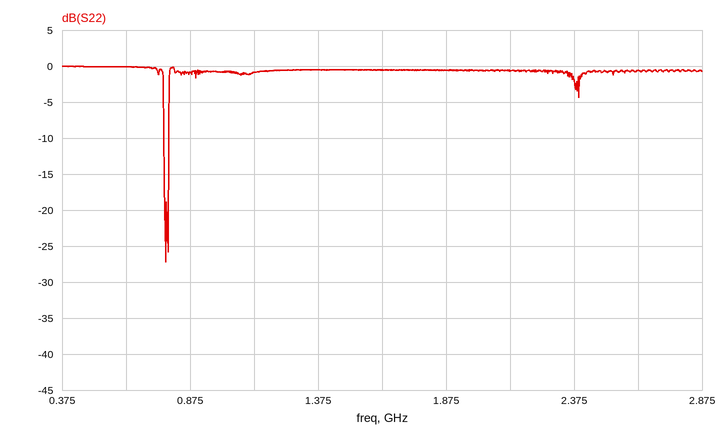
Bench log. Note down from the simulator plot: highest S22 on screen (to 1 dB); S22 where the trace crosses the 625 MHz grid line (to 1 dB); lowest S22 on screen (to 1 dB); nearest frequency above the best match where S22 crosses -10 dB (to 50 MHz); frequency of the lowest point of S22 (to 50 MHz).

0 dB
0 dB
-27 dB
800 MHz
800 MHz
